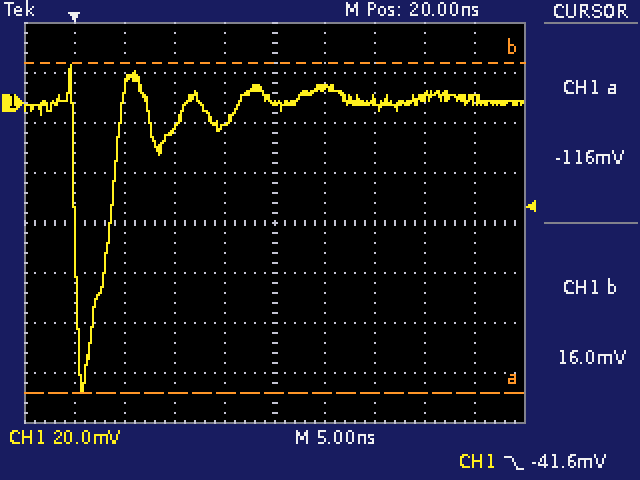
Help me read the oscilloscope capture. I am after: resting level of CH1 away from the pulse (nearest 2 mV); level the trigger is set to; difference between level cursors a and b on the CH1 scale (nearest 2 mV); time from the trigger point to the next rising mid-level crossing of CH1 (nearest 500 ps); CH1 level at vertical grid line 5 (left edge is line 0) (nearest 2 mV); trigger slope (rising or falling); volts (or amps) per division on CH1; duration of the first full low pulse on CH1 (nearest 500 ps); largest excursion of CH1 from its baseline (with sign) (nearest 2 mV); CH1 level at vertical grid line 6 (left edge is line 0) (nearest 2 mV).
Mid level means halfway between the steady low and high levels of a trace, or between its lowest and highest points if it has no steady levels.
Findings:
0 mV
-41.6 mV
132 mV
3.5 ns
0 mV
falling
20 mV
3.5 ns
-116 mV
6 mV
